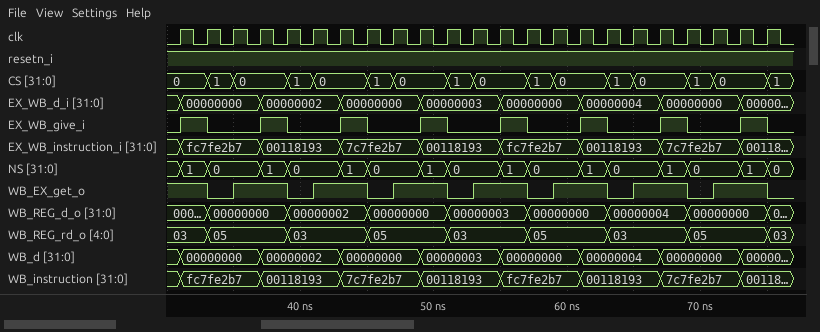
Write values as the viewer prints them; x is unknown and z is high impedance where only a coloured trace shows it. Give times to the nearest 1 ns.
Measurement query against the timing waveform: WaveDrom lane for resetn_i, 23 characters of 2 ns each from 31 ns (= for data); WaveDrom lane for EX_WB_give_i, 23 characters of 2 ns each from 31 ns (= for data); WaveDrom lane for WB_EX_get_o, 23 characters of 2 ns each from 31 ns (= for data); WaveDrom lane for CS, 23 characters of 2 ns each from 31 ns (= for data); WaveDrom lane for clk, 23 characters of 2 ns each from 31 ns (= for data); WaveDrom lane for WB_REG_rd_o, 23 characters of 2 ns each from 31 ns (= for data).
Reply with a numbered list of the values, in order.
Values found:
1. {name: 'resetn_i', wave: '1......................'}
2. {name: 'EX_WB_give_i', wave: '10.10.10.10.10.10.10.10'}
3. {name: 'WB_EX_get_o', wave: '101.01.01.01.01.01.01.0'}
4. {name: 'CS', wave: '===.==.==.==.==.==.==.=', data: '0 1 0 1 0 1 0 1 0 1 0 1 0 1 0 1'}
5. {name: 'clk', wave: 'p......................'}
6. {name: 'WB_REG_rd_o', wave: '==..=..=..=..=..=..=..=', data: '03 05 03 05 03 05 03 05 03'}
